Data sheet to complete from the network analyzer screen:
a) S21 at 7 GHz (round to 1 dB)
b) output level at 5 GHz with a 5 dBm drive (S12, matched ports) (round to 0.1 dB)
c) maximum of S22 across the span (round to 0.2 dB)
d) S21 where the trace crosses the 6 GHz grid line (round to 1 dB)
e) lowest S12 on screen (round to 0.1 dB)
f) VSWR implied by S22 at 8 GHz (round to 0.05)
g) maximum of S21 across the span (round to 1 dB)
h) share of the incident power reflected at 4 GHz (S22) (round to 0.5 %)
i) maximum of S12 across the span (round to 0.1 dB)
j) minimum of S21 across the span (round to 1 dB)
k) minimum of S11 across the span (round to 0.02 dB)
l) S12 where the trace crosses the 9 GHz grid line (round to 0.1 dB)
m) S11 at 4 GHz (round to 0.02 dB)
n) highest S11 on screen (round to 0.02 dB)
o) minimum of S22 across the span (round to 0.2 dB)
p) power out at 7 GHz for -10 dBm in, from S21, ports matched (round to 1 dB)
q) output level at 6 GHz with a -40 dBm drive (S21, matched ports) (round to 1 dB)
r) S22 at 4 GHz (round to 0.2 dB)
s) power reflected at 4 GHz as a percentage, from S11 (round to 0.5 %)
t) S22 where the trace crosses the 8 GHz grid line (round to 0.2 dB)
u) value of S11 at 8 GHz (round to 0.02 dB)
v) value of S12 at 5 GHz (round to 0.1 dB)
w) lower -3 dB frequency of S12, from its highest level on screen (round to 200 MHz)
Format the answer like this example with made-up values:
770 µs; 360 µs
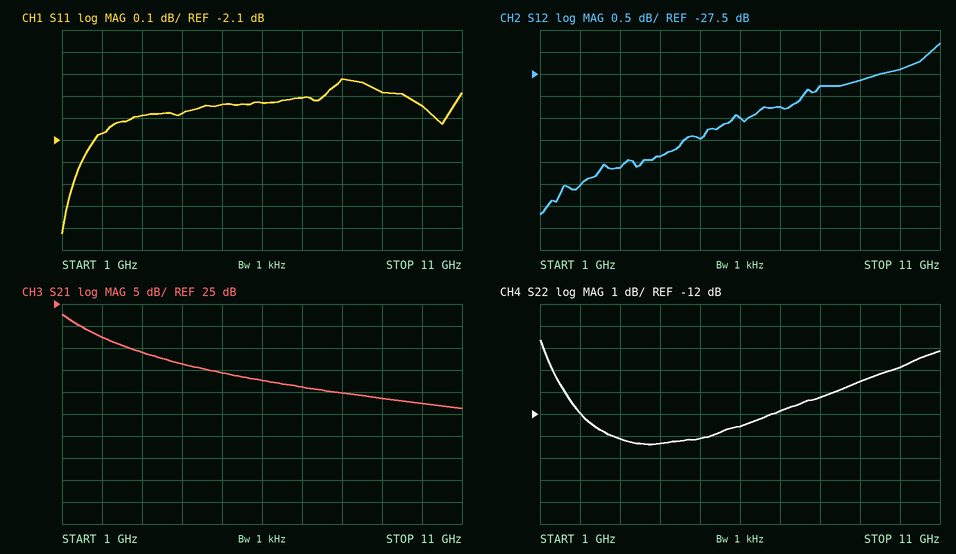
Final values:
6 dB; -24.0 dBm; -8.6 dB; 8 dB; -30.7 dB; 1.75; 23 dB; 4.5 %; -26.8 dB; 1 dB; -2.52 dB; -27.6 dB; -1.98 dB; -1.82 dB; -13.4 dB; -4 dBm; -32 dBm; -13.4 dB; 63.5 %; -11.2 dB; -1.82 dB; -29.0 dB; 2.4 GHz
